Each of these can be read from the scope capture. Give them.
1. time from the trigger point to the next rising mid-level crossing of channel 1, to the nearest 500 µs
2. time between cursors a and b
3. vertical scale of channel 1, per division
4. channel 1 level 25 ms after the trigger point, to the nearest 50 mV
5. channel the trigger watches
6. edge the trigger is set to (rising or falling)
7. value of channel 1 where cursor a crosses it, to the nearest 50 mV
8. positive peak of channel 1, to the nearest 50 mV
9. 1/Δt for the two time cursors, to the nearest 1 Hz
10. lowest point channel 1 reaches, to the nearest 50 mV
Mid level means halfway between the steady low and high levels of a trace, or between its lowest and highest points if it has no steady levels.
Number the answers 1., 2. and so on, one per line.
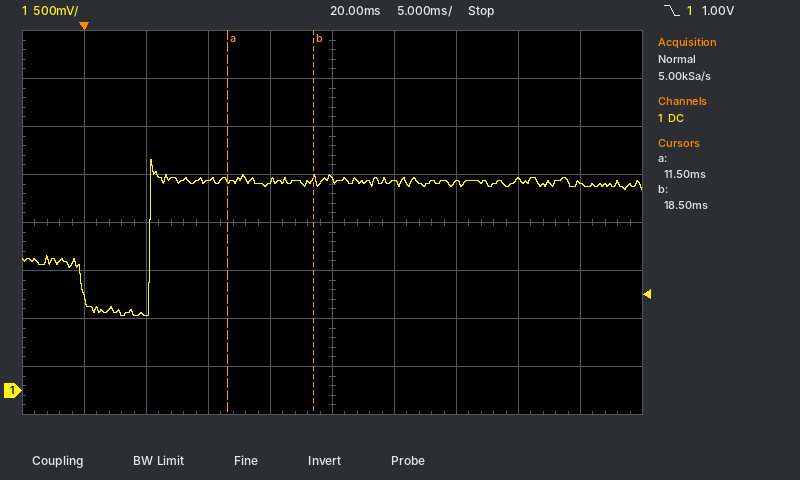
1. 5.5 ms
2. 7.0 ms
3. 500 mV
4. 2.20 V
5. channel 1
6. falling
7. 2.20 V
8. 2.40 V
9. 143 Hz
10. 800 mV
